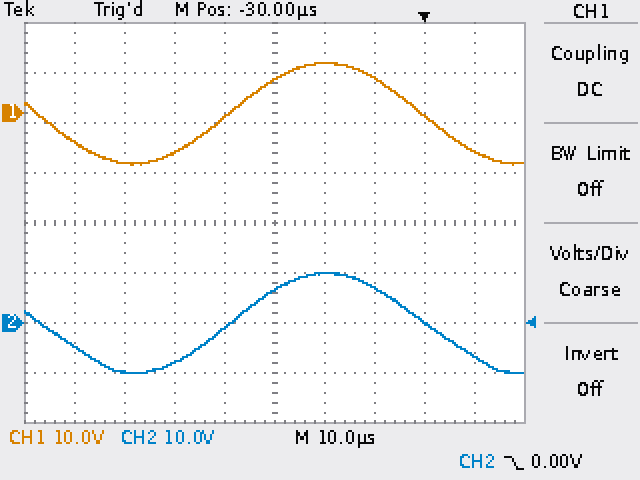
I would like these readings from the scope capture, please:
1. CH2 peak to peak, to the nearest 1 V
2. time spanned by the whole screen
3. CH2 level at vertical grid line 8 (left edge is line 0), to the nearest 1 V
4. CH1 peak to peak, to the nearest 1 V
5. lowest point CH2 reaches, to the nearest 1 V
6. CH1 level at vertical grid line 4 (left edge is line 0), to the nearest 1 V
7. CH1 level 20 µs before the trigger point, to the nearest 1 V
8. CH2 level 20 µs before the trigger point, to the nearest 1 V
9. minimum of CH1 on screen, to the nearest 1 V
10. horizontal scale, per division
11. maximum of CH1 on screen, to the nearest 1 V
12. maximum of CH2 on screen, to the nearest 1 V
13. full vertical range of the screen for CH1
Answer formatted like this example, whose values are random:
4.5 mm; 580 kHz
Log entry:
20 V; 100 µs; 0 V; 20 V; -10 V; -1 V; 10 V; 10 V; -10 V; 10 µs; 10 V; 10 V; 80 V
